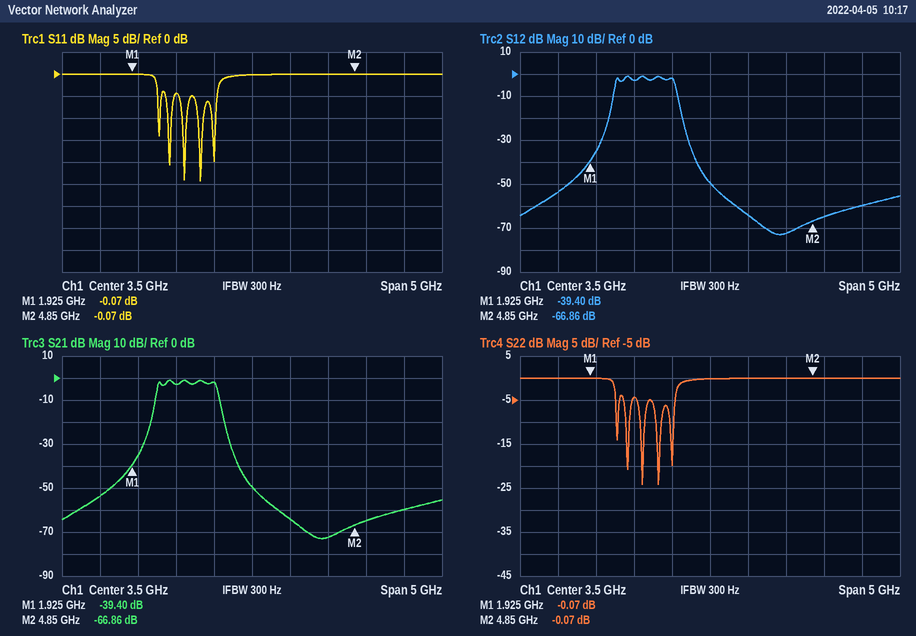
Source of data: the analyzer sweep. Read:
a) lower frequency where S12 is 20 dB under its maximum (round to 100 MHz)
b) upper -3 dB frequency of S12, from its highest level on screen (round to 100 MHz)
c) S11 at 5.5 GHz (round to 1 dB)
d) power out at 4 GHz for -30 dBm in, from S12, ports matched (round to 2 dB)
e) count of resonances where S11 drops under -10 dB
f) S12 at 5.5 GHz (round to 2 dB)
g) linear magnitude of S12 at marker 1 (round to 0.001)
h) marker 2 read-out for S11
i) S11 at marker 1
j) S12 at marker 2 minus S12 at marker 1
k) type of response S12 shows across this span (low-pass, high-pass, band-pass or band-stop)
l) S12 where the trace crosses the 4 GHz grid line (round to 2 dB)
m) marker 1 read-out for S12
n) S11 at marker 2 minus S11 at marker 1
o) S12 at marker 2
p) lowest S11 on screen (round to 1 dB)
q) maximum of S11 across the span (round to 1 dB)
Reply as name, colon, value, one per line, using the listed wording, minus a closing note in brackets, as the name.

lower frequency where S12 is 20 dB under its maximum: 2.2 GHz
upper -3 dB frequency of S12, from its highest level on screen: 3.0 GHz
S11 at 5.5 GHz: 0 dB
power out at 4 GHz for -30 dBm in, from S12, ports matched: -94 dBm
count of resonances where S11 drops under -10 dB: 5
S12 at 5.5 GHz: -60 dB
linear magnitude of S12 at marker 1: 0.011
marker 2 read-out for S11: -0.07 dB
S11 at marker 1: -0.07 dB
S12 at marker 2 minus S12 at marker 1: -27.46 dB
type of response S12 shows across this span: band-pass
S12 where the trace crosses the 4 GHz grid line: -64 dB
marker 1 read-out for S12: -39.40 dB
S11 at marker 2 minus S11 at marker 1: 0.00 dB
S12 at marker 2: -66.86 dB
lowest S11 on screen: -24 dB
maximum of S11 across the span: 0 dB
